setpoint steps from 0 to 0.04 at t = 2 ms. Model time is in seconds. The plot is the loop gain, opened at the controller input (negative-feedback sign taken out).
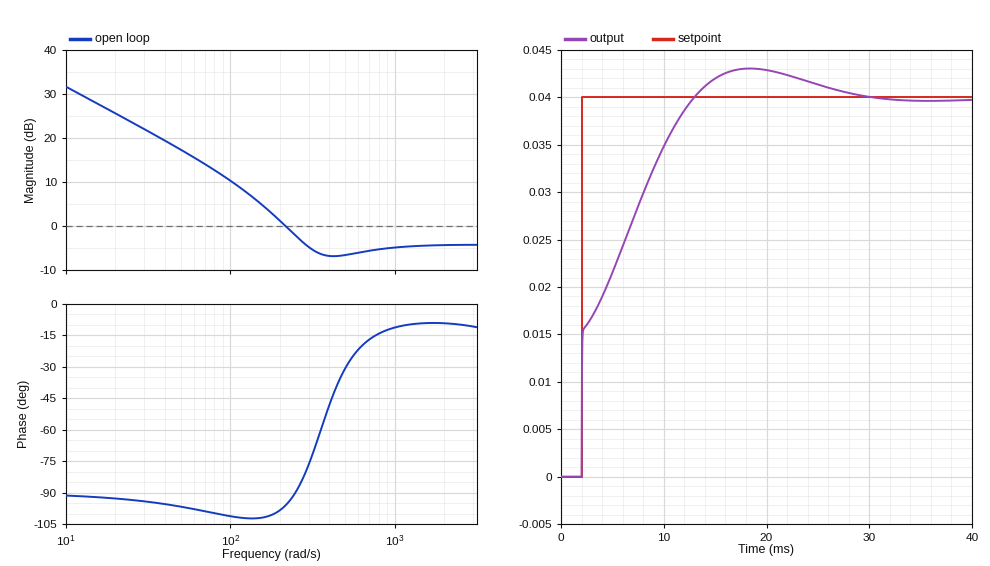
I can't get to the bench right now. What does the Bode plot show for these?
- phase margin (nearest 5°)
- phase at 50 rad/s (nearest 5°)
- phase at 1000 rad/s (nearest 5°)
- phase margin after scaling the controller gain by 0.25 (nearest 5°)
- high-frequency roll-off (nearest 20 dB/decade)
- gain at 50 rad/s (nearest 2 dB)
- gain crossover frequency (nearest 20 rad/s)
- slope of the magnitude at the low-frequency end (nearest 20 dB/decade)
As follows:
85°
-95°
-10°
80°
0 dB/decade
18 dB
220 rad/s
-20 dB/decade
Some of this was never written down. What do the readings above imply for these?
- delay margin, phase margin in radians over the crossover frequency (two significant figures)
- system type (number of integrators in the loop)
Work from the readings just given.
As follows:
0.0067 s
1
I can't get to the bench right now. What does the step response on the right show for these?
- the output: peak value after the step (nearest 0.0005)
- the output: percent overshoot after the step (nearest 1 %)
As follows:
0.0430
8 %
